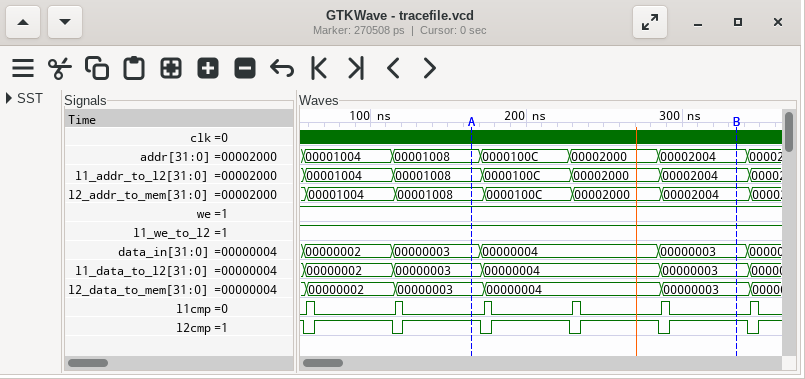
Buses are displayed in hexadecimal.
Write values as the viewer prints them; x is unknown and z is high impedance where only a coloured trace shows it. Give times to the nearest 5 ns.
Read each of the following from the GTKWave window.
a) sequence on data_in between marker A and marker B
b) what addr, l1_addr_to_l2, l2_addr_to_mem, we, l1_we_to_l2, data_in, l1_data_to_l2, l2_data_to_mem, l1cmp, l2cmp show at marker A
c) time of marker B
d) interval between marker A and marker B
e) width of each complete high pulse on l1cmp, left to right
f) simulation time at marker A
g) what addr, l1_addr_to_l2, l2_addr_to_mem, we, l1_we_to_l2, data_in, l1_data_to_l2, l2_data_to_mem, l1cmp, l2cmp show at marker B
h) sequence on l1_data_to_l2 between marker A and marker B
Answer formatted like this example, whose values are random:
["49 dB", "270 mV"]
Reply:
["00000003, 00000004, 00000003", "addr=00001008, l1_addr_to_l2=00001008, l2_addr_to_mem=00001008, we=1, l1_we_to_l2=1, data_in=00000003, l1_data_to_l2=00000003, l2_data_to_mem=00000003, l1cmp=0, l2cmp=1", "335 ns", "170 ns", "5 ns, 5 ns, 5 ns, 5 ns, 5 ns, 5 ns", "165 ns", "addr=00002004, l1_addr_to_l2=00002004, l2_addr_to_mem=00002004, we=1, l1_we_to_l2=1, data_in=00000003, l1_data_to_l2=00000003, l2_data_to_mem=00000003, l1cmp=0, l2cmp=1", "00000003, 00000004, 00000003"]
